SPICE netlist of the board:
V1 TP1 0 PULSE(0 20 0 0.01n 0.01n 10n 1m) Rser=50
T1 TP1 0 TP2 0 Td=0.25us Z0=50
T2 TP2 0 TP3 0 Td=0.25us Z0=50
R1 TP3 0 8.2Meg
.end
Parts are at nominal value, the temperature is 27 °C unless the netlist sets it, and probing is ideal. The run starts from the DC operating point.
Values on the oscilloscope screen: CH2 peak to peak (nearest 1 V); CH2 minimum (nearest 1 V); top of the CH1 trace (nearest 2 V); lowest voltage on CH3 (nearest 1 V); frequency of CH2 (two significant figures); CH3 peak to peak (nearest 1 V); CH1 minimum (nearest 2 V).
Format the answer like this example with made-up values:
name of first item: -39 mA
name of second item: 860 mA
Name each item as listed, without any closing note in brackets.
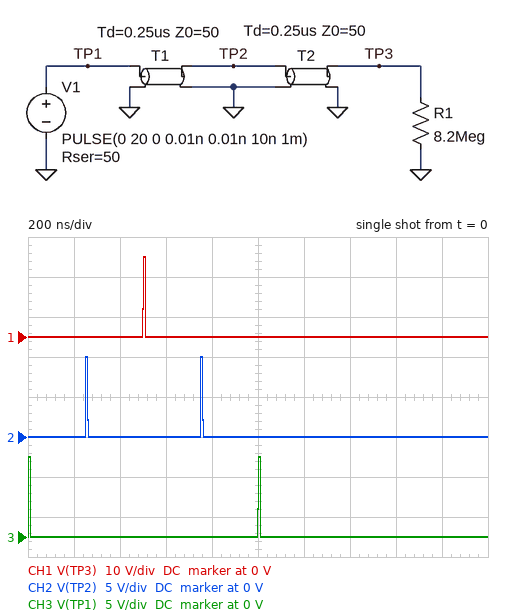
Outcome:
CH2 peak to peak: 10 V
CH2 minimum: 0 V
top of the CH1 trace: 20 V
lowest voltage on CH3: 0 V
frequency of CH2: 2.0 MHz
CH3 peak to peak: 10 V
CH1 minimum: 0 V
